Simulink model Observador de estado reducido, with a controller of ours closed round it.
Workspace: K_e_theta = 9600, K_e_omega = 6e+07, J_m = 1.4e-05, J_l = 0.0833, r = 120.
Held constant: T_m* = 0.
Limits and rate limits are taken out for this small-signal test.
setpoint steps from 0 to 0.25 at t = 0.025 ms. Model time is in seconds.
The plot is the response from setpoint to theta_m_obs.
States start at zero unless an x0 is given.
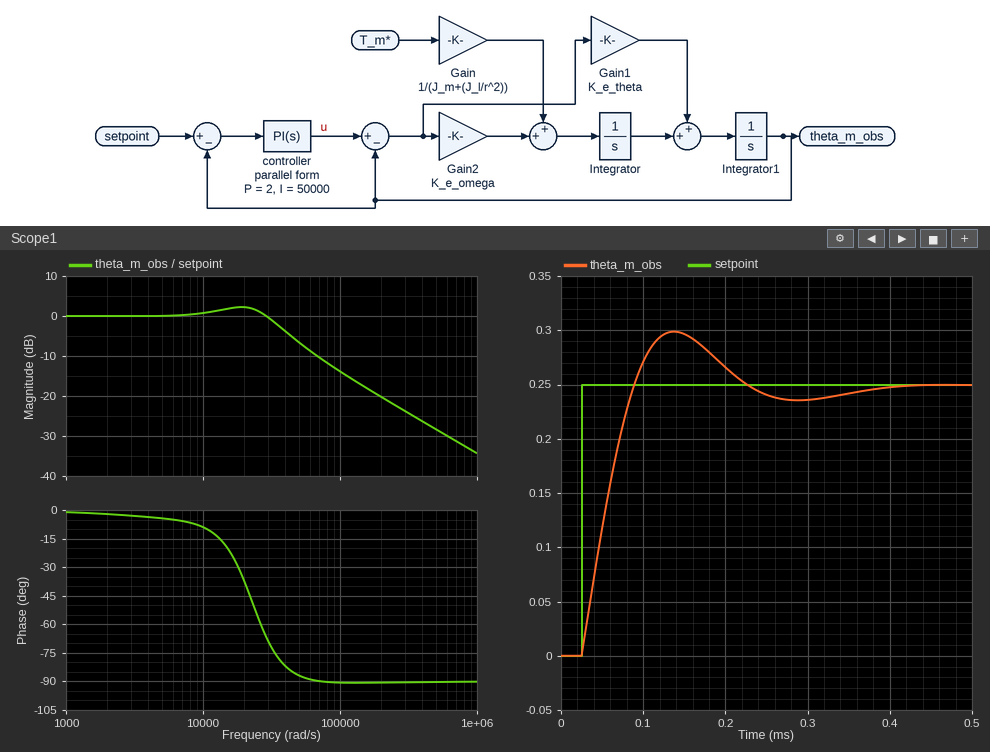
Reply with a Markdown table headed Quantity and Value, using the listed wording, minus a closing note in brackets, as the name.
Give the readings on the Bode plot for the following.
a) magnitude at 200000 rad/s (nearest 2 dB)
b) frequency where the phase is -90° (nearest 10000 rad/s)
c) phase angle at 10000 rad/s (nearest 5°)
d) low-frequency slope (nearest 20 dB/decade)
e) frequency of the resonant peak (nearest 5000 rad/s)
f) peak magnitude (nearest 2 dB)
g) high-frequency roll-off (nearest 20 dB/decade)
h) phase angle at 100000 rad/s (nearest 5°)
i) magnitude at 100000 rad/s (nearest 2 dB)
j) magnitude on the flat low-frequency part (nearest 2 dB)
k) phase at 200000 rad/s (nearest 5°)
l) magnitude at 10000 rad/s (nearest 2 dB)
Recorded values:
| Quantity | Value |
|---|---|
| magnitude at 200000 rad/s | -20 dB |
| frequency where the phase is -90° | 70000 rad/s |
| phase angle at 10000 rad/s | -10° |
| low-frequency slope | 0 dB/decade |
| frequency of the resonant peak | 20000 rad/s |
| peak magnitude | 2 dB |
| high-frequency roll-off | -20 dB/decade |
| phase angle at 100000 rad/s | -90° |
| magnitude at 100000 rad/s | -14 dB |
| magnitude on the flat low-frequency part | 0 dB |
| phase at 200000 rad/s | -90° |
| magnitude at 10000 rad/s | 0 dB |
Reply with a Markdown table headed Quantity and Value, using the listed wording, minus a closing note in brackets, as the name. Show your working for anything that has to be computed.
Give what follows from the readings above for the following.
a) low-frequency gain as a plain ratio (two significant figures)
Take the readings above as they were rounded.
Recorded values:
| Quantity | Value |
|---|---|
| low-frequency gain as a plain ratio | 10^(0 / 20) = 1.0 |
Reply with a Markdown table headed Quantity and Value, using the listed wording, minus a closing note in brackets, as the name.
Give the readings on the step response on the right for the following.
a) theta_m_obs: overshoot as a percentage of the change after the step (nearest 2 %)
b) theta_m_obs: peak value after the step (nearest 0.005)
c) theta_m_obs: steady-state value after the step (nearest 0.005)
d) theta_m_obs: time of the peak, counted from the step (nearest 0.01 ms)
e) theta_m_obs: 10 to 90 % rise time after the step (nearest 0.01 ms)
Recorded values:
| Quantity | Value |
|---|---|
| theta_m_obs: overshoot as a percentage of the change after the step | 20 % |
| theta_m_obs: peak value after the step | 0.300 |
| theta_m_obs: steady-state value after the step | 0.250 |
| theta_m_obs: time of the peak, counted from the step | 0.11 ms |
| theta_m_obs: 10 to 90 % rise time after the step | 0.05 ms |
